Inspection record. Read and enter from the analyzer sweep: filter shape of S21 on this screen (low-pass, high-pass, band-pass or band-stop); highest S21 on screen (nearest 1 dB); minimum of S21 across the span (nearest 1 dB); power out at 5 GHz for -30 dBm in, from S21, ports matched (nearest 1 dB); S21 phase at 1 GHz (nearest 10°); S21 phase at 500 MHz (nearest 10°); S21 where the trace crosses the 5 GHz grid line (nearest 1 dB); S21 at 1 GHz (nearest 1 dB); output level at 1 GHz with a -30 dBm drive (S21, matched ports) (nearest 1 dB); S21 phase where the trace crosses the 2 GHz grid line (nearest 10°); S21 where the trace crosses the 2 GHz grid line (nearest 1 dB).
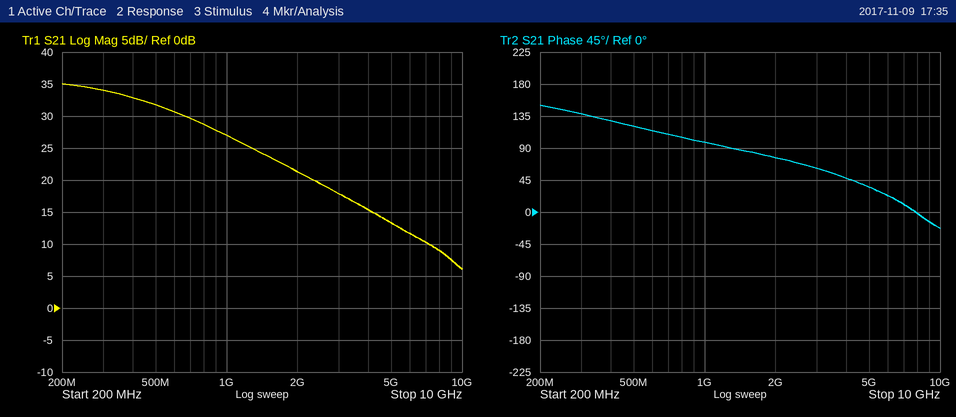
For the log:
low-pass
35 dB
6 dB
-17 dBm
100°
120°
13 dB
27 dB
-3 dBm
80°
21 dB
